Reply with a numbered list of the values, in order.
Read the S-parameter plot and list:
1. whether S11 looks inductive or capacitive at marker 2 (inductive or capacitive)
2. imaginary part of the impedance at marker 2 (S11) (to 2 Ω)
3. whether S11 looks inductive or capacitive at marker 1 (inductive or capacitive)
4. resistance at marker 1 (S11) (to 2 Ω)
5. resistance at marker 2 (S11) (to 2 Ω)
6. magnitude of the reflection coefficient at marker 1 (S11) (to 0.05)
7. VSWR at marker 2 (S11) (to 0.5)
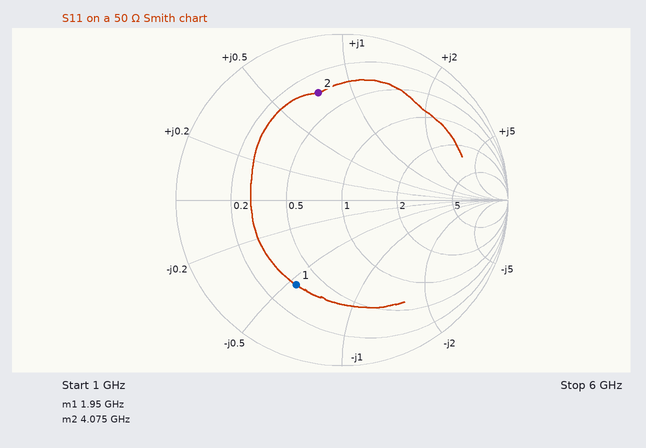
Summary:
1. inductive
2. +38 Ω
3. capacitive
4. 18 Ω
5. 16 Ω
6. 0.60
7. 5.0
